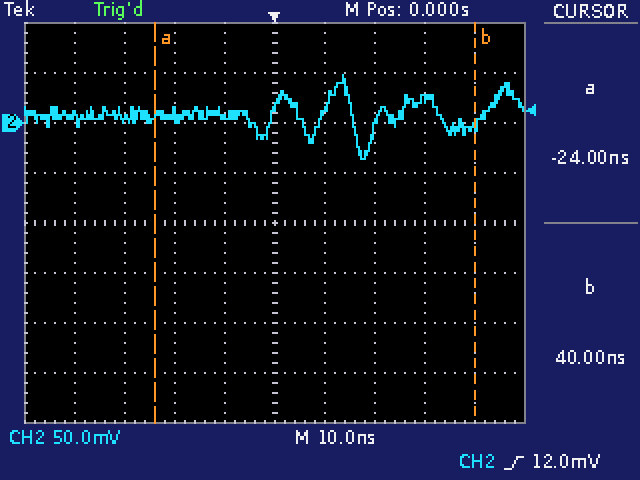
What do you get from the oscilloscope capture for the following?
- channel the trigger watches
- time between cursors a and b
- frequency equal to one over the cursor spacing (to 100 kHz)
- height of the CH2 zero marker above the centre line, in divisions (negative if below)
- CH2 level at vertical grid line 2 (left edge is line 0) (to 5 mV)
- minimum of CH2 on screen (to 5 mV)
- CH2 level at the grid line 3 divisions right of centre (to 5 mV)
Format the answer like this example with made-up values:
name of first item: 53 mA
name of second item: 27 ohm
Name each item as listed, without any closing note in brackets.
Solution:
channel the trigger watches: CH2
time between cursors a and b: 64 ns
frequency equal to one over the cursor spacing: 15.6 MHz
height of the CH2 zero marker above the centre line, in divisions: +2.0 div
CH2 level at vertical grid line 2 (left edge is line 0): 5 mV
minimum of CH2 on screen: -35 mV
CH2 level at the grid line 3 divisions right of centre: 25 mV
